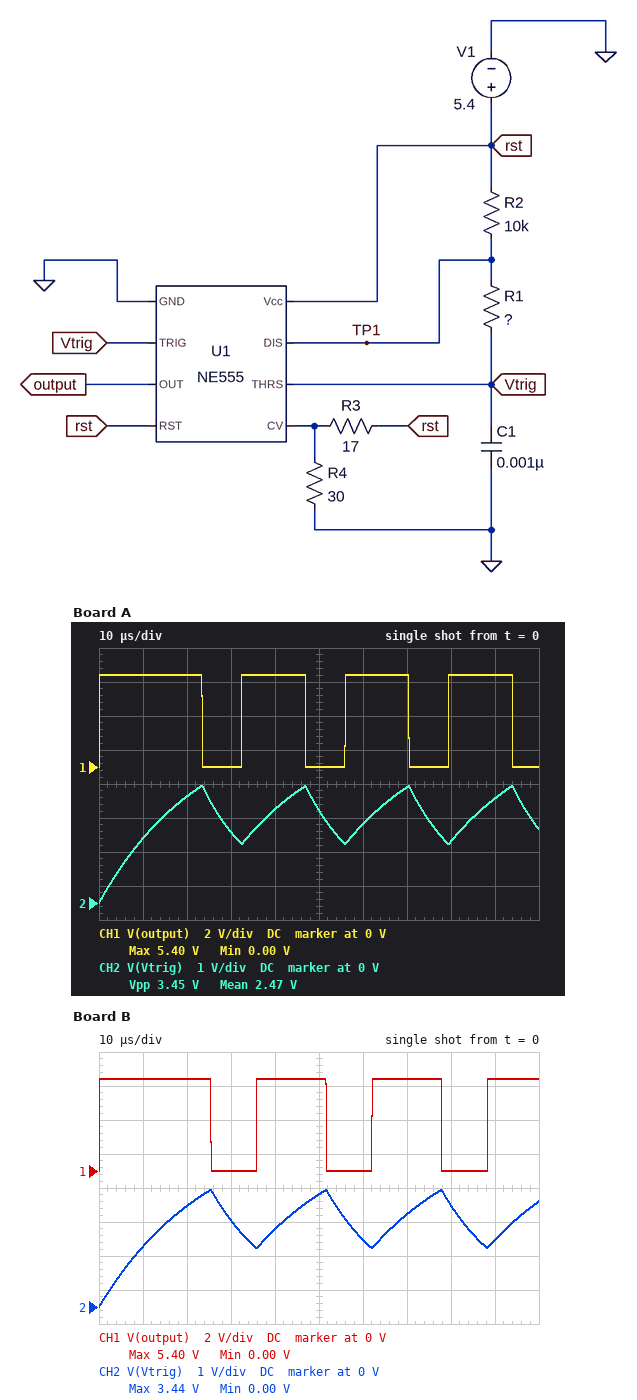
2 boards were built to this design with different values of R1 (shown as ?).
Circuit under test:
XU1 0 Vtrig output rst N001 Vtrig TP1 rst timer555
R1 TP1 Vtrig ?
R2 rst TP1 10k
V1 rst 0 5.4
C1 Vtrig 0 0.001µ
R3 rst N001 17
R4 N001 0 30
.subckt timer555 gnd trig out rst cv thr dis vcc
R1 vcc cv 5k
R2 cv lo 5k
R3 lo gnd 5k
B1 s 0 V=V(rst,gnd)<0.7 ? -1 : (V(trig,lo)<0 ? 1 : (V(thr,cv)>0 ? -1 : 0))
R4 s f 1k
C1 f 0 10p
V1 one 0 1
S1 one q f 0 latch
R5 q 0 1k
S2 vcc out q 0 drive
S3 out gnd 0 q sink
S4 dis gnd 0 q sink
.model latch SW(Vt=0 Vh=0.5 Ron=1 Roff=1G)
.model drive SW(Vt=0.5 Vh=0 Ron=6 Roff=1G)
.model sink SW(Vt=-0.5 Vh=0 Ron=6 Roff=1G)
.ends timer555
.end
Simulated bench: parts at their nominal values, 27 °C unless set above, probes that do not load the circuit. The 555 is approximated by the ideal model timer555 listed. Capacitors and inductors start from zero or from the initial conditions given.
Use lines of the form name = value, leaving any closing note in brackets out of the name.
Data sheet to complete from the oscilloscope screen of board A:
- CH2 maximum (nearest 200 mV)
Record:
CH2 maximum = 3.4 V
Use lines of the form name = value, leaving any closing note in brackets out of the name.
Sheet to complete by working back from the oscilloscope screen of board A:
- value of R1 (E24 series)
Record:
value of R1 = 13 kΩ
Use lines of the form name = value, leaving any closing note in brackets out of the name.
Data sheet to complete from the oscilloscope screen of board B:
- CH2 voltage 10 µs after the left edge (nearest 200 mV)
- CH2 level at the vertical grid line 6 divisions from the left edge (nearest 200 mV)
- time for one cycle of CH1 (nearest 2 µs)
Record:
CH2 voltage 10 µs after the left edge = 1.8 V
CH2 level at the vertical grid line 6 divisions from the left edge = 2.0 V
time for one cycle of CH1 = 26 µs
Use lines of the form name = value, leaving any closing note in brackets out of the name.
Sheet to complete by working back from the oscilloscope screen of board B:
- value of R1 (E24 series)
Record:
value of R1 = 15 kΩ
